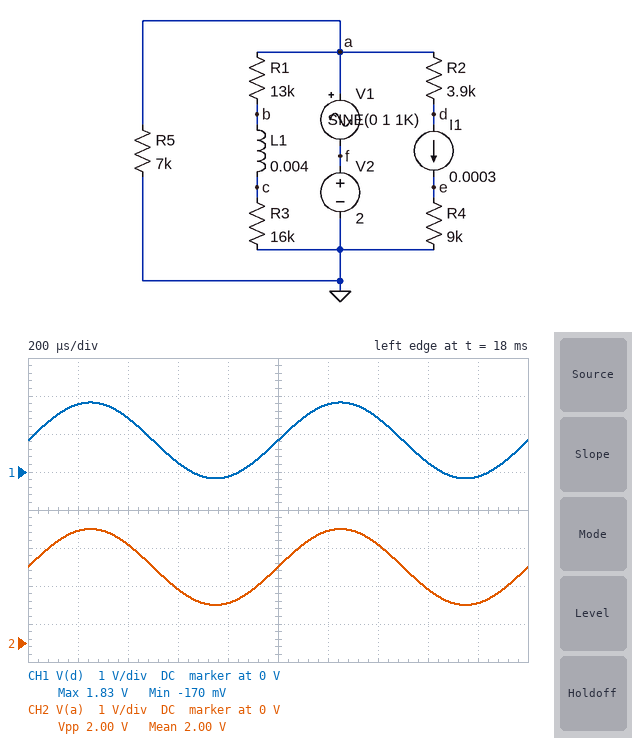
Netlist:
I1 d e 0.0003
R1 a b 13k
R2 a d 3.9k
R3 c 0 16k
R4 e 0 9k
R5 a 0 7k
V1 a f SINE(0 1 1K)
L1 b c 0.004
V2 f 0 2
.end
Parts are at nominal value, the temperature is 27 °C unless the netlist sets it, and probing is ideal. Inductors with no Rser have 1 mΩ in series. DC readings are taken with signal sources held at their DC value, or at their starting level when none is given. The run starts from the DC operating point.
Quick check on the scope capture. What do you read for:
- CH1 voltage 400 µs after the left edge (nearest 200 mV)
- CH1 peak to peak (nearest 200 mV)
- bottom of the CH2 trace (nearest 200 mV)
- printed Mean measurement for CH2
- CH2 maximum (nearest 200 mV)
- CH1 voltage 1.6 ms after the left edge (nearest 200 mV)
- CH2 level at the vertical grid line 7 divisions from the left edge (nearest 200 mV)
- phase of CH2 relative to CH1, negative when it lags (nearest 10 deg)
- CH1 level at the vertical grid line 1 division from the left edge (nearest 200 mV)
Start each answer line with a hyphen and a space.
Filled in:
- 1.4 V
- 2.0 V
- 1.0 V
- 2.00 V
- 3.0 V
- 200 mV
- 2.6 V
- 0 deg
- 1.8 V
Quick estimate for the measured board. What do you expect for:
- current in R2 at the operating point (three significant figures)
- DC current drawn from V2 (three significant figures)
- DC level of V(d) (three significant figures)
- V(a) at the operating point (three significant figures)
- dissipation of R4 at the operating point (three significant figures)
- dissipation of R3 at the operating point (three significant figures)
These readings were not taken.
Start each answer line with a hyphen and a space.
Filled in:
- 300 µA
- 655 µA
- 830 mV
- 2.00 V
- 810 µW
- 76.1 µW
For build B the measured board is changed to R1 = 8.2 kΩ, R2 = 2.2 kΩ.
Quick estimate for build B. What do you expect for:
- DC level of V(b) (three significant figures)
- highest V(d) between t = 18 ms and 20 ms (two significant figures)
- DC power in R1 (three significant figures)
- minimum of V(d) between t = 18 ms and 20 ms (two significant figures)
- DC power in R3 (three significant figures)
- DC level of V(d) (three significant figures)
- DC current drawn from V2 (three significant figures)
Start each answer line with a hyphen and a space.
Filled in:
- 1.32 V
- 2.3 V
- 56.0 µW
- 340 mV
- 109 µW
- 1.34 V
- 668 µA
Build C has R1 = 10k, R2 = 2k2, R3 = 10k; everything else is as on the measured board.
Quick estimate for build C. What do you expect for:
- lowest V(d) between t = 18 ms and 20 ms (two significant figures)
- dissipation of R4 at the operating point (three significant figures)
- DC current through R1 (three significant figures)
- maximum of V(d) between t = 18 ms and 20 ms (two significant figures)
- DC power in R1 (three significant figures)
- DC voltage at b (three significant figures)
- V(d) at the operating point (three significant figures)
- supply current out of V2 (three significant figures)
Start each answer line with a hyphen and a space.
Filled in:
- 340 mV
- 810 µW
- 100 µA
- 2.3 V
- 100 µW
- 1.00 V
- 1.34 V
- 686 µA
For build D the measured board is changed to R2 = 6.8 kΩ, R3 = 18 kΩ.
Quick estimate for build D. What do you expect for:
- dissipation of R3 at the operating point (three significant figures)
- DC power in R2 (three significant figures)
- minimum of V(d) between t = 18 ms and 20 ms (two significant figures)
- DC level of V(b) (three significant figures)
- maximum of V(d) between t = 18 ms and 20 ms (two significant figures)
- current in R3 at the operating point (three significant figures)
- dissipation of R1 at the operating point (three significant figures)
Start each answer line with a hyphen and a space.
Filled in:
- 74.9 µW
- 612 µW
- -1.0 V
- 1.16 V
- 960 mV
- 64.5 µA
- 54.1 µW
